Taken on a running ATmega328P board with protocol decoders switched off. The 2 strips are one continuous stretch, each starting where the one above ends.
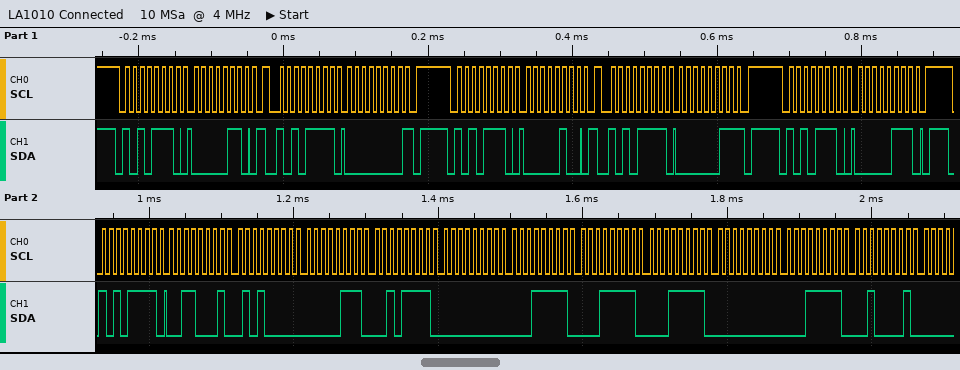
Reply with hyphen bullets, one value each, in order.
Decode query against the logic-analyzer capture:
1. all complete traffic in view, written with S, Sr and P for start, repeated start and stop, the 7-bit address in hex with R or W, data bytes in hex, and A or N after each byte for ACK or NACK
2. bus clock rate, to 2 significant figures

- S 57W A 06 A Sr 57R A 00 N P S 57W A 04 A Sr 57R A 03 N P S 57W A 07 A P S 57R A 31 A 50 A 07 A 2F A 00 A 1F A 1F A 1F A 00 A 1F A 21 A
- 100 kHz
